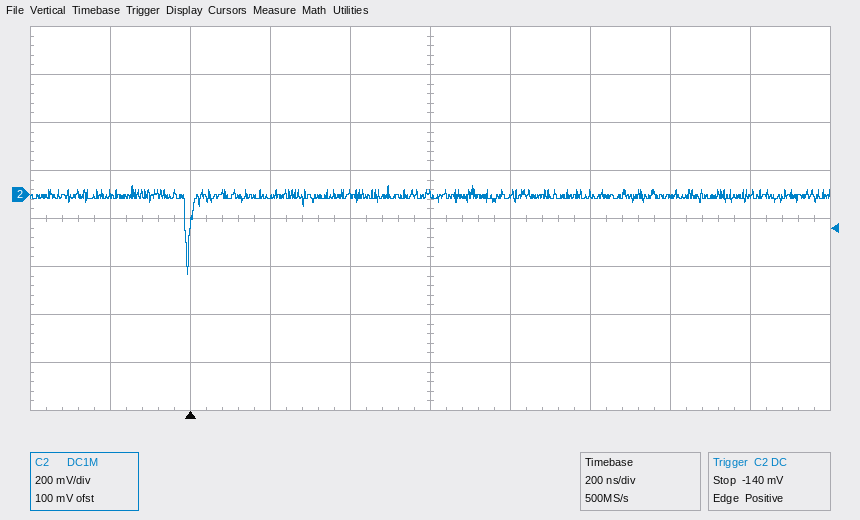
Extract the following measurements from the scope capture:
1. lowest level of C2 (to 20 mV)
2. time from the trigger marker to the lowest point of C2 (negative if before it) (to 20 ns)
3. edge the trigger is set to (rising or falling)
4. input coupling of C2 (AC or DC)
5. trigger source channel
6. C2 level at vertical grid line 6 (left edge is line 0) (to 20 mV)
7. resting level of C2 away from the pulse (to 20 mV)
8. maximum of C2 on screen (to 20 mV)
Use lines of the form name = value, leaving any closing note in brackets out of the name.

lowest level of C2 = -340 mV
time from the trigger marker to the lowest point of C2 (negative if before it) = 0 ns
edge the trigger is set to = rising
input coupling of C2 = DC
trigger source channel = C2
C2 level at vertical grid line 6 (left edge is line 0) = 0 mV
resting level of C2 away from the pulse = 0 mV
maximum of C2 on screen = 40 mV
